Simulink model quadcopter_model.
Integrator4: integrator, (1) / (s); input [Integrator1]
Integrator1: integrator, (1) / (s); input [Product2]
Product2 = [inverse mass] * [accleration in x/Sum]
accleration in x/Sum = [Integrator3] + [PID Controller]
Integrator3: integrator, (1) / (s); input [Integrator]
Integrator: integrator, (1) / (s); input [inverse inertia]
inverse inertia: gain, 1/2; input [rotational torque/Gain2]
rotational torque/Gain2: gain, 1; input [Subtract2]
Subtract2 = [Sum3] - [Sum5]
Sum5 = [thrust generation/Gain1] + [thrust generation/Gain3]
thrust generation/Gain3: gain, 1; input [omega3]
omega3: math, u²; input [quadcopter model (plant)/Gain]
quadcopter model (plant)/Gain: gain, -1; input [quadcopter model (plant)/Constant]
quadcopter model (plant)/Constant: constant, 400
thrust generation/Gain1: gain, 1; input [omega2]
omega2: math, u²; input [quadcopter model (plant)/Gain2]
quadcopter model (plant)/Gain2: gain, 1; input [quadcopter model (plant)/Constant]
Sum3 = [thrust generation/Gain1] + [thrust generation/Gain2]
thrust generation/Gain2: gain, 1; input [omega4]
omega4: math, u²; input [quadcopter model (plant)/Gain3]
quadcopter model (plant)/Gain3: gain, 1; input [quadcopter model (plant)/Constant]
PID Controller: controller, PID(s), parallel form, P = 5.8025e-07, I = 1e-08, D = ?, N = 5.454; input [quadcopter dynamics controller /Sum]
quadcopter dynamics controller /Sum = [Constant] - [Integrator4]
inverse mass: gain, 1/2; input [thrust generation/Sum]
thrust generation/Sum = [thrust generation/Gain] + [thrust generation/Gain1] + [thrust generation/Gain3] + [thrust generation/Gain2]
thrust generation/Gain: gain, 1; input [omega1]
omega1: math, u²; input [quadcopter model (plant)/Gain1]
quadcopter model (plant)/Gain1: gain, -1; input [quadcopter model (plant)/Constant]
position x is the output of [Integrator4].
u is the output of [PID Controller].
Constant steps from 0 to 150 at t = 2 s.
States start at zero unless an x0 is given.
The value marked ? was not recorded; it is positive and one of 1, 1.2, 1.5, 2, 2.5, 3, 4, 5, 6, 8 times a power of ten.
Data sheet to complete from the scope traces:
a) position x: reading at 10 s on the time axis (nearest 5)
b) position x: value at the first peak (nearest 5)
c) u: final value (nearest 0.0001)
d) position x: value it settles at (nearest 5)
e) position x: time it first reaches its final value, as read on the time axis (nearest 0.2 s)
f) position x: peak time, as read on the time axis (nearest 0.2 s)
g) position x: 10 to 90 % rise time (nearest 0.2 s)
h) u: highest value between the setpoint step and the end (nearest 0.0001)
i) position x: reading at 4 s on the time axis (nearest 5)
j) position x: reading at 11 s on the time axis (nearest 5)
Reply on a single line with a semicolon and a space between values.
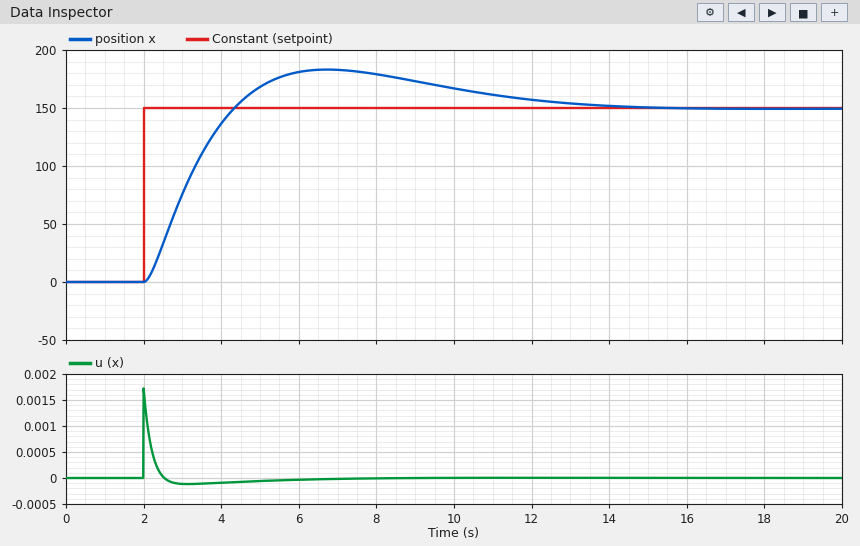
165; 185; 0.0000; 150; 4.4 s; 6.8 s; 1.6 s; 0.0017; 135; 160
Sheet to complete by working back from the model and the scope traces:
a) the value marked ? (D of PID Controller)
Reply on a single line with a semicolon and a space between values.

2e-06
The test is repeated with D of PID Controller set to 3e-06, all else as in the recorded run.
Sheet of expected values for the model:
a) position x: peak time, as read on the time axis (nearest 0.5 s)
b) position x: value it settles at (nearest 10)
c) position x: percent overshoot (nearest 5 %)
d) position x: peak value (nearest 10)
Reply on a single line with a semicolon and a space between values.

6.0 s; 150; 15 %; 170
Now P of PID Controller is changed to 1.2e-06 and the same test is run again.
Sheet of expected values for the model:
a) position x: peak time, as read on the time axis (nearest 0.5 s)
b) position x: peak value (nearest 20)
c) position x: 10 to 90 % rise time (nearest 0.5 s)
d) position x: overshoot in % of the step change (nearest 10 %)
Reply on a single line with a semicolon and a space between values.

5.5 s; 200; 1.5 s; 30 %
